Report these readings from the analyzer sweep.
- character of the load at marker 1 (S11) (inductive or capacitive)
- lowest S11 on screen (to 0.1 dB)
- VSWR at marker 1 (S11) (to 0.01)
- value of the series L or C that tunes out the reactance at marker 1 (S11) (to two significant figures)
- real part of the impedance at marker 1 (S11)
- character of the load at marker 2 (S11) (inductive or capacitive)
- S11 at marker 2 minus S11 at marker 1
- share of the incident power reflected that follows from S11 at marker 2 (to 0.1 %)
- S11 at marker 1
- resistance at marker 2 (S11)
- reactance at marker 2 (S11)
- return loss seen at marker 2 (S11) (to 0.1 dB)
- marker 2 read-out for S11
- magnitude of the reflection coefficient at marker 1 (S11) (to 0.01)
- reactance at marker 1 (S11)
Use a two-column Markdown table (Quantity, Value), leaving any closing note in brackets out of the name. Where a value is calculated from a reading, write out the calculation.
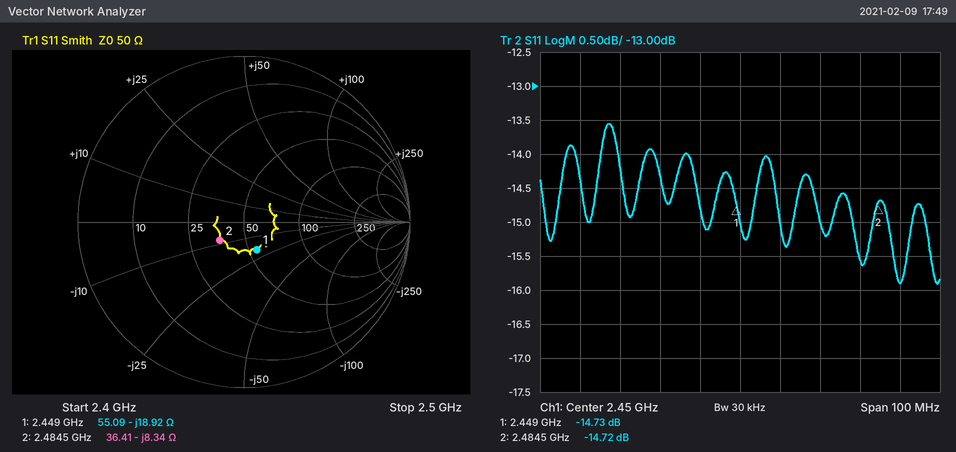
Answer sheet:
| Quantity | Value |
|---|---|
| character of the load at marker 1 (S11) | capacitive |
| lowest S11 on screen | -15.9 dB |
| VSWR at marker 1 (S11) | (1 + 0.1834)/(1 − 0.1834) ≈ 1.45 |
| value of the series L or C that tunes out the reactance at marker 1 (S11) | L = 18.92 Ω/(2π × 2.449 GHz) ≈ 1.2 nH |
| real part of the impedance at marker 1 | 55.09 Ω |
| character of the load at marker 2 (S11) | capacitive |
| S11 at marker 2 minus S11 at marker 1 | -14.72 − (-14.73) = 0.01 dB |
| share of the incident power reflected that follows from S11 at marker 2 | 10^(-14.72/10) ≈ 3.4 % |
| S11 at marker 1 | -14.73 dB |
| resistance at marker 2 | 36.41 Ω |
| reactance at marker 2 | -8.34 Ω |
| return loss seen at marker 2 (S11) | 14.7 dB |
| marker 2 read-out for S11 | -14.72 dB |
| magnitude of the reflection coefficient at marker 1 (S11) | 0.18 |
| reactance at marker 1 | -18.92 Ω |
